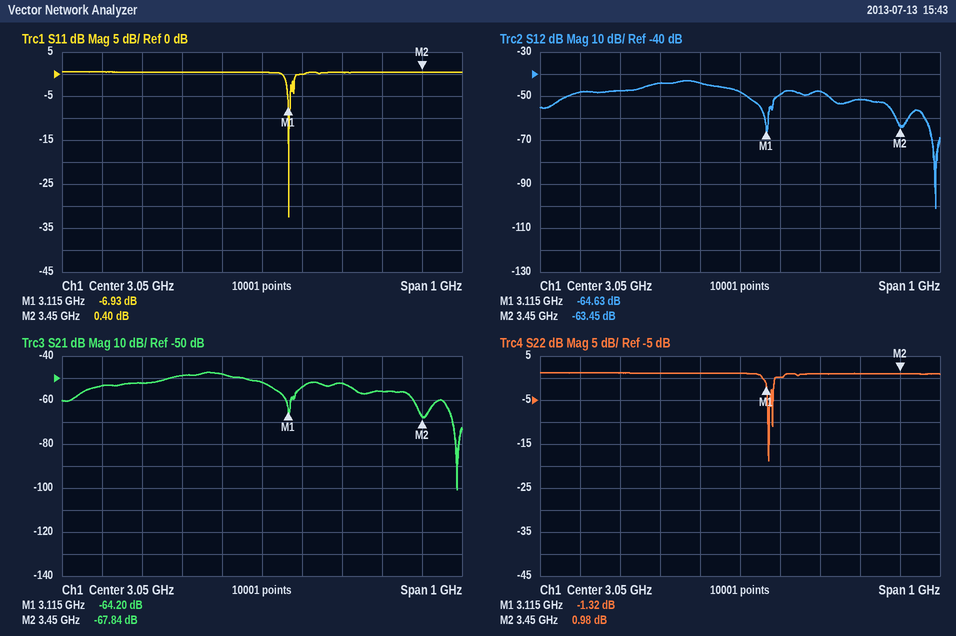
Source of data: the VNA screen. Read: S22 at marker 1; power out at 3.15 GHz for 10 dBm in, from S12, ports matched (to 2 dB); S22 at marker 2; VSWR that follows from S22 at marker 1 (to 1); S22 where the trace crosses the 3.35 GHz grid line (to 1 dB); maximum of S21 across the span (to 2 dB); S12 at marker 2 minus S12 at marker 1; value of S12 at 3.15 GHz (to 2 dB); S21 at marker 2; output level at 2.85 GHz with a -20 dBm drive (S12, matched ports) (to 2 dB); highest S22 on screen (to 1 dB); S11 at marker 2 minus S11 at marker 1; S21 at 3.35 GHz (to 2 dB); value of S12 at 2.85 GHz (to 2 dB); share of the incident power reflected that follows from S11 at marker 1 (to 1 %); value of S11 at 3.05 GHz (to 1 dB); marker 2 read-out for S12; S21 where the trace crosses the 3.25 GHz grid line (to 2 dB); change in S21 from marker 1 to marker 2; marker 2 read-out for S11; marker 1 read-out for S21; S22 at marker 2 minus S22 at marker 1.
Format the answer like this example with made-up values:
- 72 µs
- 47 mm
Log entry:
- -1.32 dB
- -40 dBm
- 0.98 dB
- 13
- 1 dB
- -48 dB
- 1.18 dB
- -50 dB
- -67.84 dB
- -64 dBm
- 1 dB
- 7.33 dB
- -56 dB
- -44 dB
- 20 %
- 0 dB
- -63.45 dB
- -52 dB
- -3.64 dB
- 0.40 dB
- -64.20 dB
- 2.30 dB
